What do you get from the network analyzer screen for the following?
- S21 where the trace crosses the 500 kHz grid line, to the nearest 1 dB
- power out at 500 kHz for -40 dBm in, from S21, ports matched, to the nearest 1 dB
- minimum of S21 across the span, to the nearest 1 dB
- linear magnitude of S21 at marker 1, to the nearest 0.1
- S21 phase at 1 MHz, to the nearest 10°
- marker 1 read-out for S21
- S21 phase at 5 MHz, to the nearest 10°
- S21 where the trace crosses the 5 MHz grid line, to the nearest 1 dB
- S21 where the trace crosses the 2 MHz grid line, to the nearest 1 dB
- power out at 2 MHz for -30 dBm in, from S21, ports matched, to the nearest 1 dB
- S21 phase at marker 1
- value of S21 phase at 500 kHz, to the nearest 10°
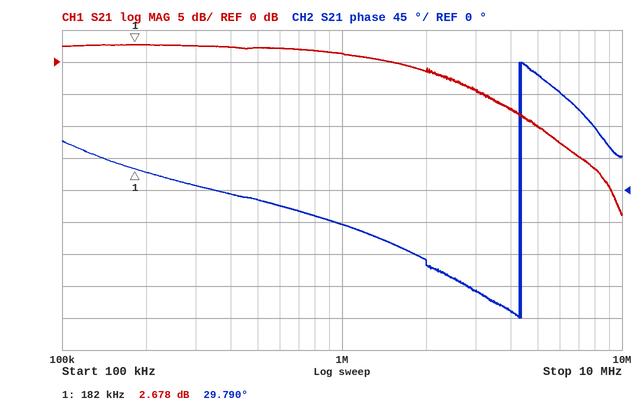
2 dB
-38 dBm
-24 dB
1.4
-50°
2.678 dB
160°
-10 dB
-1 dB
-31 dBm
29.790°
-10°
